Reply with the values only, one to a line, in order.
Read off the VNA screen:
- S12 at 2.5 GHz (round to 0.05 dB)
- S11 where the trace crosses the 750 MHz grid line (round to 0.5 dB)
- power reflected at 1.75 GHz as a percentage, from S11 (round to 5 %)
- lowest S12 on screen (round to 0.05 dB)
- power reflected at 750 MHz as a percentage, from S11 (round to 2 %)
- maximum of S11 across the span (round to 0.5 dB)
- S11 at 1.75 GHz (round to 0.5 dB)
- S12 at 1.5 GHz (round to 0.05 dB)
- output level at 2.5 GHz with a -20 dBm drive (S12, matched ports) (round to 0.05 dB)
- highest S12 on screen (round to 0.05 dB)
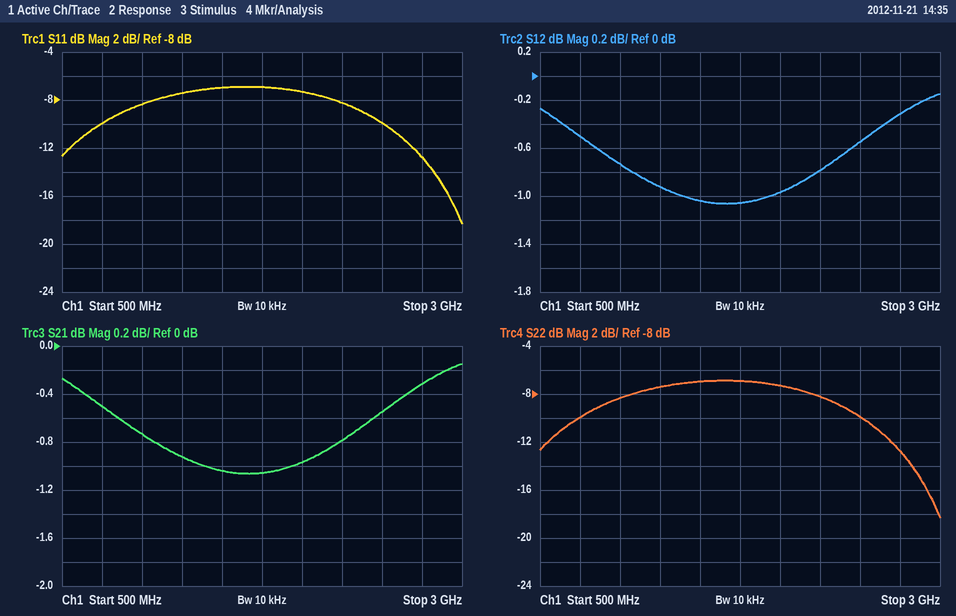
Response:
-0.55 dB
-10.0 dB
20 %
-1.05 dB
10 %
-7.0 dB
-7.0 dB
-1.05 dB
-20.55 dBm
-0.15 dB
